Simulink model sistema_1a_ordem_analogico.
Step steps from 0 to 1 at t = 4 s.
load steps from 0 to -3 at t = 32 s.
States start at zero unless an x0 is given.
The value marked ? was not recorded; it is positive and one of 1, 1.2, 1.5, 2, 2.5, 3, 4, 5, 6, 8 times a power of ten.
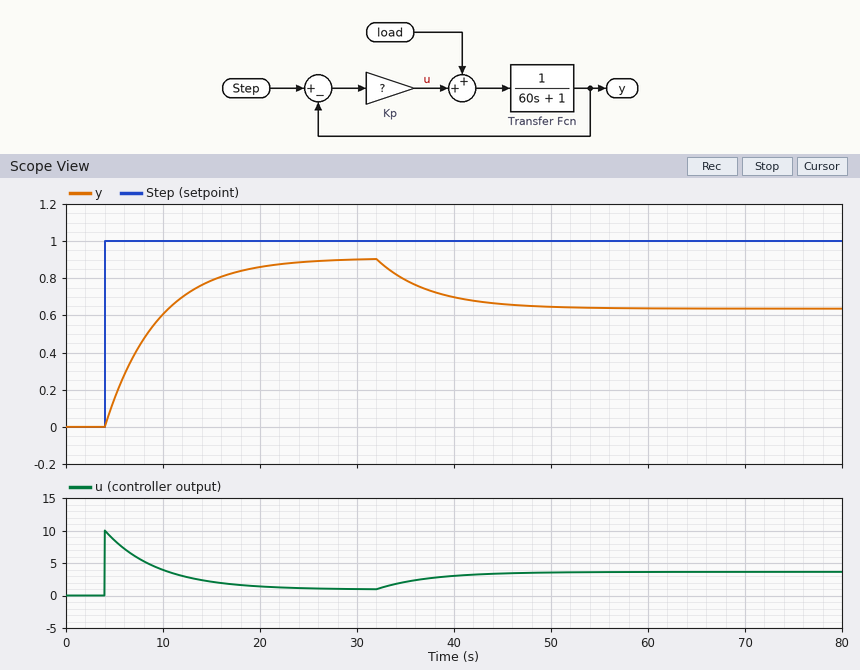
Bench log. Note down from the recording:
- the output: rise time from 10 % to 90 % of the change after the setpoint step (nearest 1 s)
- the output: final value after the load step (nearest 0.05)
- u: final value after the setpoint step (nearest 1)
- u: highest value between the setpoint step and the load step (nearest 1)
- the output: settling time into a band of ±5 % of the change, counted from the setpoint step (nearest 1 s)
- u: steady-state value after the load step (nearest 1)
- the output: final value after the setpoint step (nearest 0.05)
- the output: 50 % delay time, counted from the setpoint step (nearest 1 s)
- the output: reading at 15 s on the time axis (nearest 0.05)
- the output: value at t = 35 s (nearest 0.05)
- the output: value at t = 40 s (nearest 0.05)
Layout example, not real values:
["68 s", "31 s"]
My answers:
["12 s", "0.65", "1", "10", "16 s", "4", "0.90", "4 s", "0.80", "0.80", "0.70"]
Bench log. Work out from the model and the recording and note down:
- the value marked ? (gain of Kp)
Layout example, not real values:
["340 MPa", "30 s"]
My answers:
["10"]
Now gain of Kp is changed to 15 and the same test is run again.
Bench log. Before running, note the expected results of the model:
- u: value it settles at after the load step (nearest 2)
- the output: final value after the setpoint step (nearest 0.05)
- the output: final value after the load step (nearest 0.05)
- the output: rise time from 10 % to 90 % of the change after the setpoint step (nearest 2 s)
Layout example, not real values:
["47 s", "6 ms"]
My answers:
["4", "0.95", "0.75", "8 s"]
